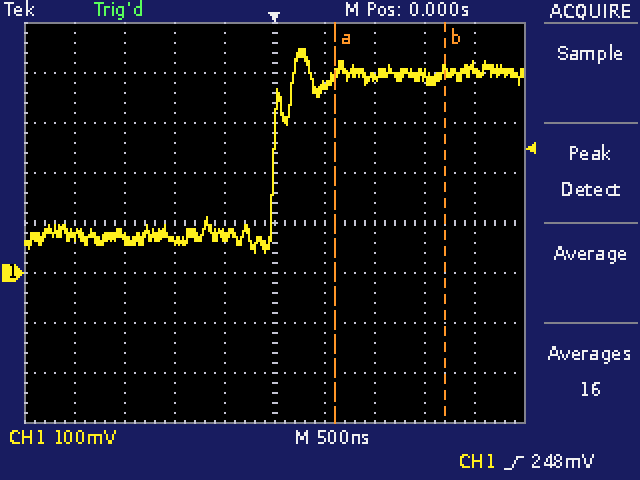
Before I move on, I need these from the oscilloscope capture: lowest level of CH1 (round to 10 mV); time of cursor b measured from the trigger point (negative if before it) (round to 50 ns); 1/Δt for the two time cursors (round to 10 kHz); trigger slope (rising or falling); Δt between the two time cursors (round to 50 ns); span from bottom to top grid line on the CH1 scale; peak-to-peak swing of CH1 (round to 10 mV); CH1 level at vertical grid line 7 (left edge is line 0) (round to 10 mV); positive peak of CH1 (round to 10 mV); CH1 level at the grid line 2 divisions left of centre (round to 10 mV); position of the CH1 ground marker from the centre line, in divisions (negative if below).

40 mV
+1.70 µs
910 kHz
rising
1.10 µs
800 mV
410 mV
390 mV
450 mV
60 mV
-1.0 div
